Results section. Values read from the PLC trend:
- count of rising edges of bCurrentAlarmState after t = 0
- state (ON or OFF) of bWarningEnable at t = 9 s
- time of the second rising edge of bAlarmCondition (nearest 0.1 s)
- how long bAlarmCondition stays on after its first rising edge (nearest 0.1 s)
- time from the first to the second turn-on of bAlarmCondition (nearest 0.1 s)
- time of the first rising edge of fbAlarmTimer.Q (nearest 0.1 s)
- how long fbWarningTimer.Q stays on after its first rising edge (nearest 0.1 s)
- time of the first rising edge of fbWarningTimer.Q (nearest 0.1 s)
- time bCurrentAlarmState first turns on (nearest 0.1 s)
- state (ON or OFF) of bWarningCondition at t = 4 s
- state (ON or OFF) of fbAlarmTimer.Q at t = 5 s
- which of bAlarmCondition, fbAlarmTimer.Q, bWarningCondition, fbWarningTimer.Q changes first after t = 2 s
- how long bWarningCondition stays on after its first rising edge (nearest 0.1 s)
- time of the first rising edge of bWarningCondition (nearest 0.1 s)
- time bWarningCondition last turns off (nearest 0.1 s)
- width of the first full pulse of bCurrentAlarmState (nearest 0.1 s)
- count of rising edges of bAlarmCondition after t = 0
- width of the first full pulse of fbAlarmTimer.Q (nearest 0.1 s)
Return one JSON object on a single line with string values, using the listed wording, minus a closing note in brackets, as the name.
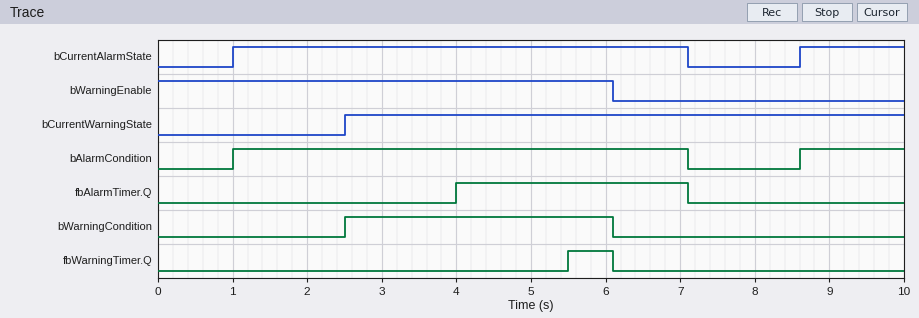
{"count of rising edges of bCurrentAlarmState after t = 0": "2", "state (ON or OFF) of bWarningEnable at t = 9 s": "OFF", "time of the second rising edge of bAlarmCondition": "8.6 s", "how long bAlarmCondition stays on after its first rising edge": "6.1 s", "time from the first to the second turn-on of bAlarmCondition": "7.6 s", "time of the first rising edge of fbAlarmTimer.Q": "4.0 s", "how long fbWarningTimer.Q stays on after its first rising edge": "0.6 s", "time of the first rising edge of fbWarningTimer.Q": "5.5 s", "time bCurrentAlarmState first turns on": "1.0 s", "state (ON or OFF) of bWarningCondition at t = 4 s": "ON", "state (ON or OFF) of fbAlarmTimer.Q at t = 5 s": "ON", "which of bAlarmCondition, fbAlarmTimer.Q, bWarningCondition, fbWarningTimer.Q changes first after t = 2 s": "bWarningCondition", "how long bWarningCondition stays on after its first rising edge": "3.6 s", "time of the first rising edge of bWarningCondition": "2.5 s", "time bWarningCondition last turns off": "6.1 s", "width of the first full pulse of bCurrentAlarmState": "6.1 s", "count of rising edges of bAlarmCondition after t = 0": "2", "width of the first full pulse of fbAlarmTimer.Q": "3.1 s"}
